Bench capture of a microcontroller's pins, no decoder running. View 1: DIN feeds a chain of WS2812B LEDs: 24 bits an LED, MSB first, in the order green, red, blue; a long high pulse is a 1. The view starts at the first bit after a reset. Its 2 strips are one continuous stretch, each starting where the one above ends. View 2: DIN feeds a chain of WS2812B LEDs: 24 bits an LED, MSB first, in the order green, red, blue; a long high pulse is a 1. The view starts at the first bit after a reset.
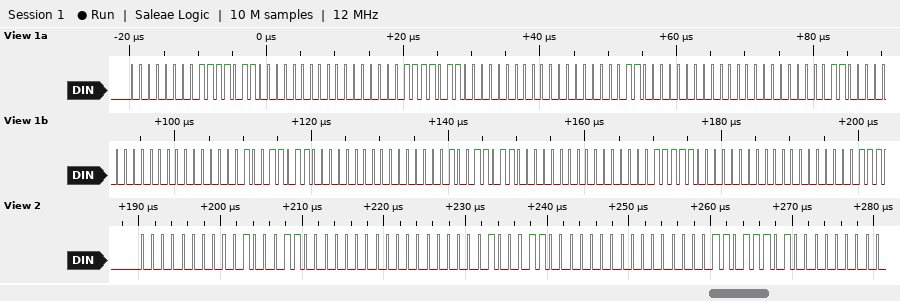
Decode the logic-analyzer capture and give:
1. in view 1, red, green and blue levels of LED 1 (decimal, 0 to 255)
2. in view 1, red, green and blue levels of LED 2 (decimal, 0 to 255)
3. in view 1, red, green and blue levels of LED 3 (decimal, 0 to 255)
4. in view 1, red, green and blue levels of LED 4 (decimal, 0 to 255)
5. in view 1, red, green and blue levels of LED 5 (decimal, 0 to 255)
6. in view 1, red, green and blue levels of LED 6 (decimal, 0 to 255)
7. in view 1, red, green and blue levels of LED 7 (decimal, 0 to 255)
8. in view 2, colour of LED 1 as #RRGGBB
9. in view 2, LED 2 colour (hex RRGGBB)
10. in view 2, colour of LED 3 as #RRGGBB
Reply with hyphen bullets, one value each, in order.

- 246, 0, 0
- 246, 0, 0
- 48, 0, 0
- 48, 0, 0
- 155, 0, 0
- 155, 0, 0
- 248, 0, 0
- #230000
- #230000
- #DD0000
